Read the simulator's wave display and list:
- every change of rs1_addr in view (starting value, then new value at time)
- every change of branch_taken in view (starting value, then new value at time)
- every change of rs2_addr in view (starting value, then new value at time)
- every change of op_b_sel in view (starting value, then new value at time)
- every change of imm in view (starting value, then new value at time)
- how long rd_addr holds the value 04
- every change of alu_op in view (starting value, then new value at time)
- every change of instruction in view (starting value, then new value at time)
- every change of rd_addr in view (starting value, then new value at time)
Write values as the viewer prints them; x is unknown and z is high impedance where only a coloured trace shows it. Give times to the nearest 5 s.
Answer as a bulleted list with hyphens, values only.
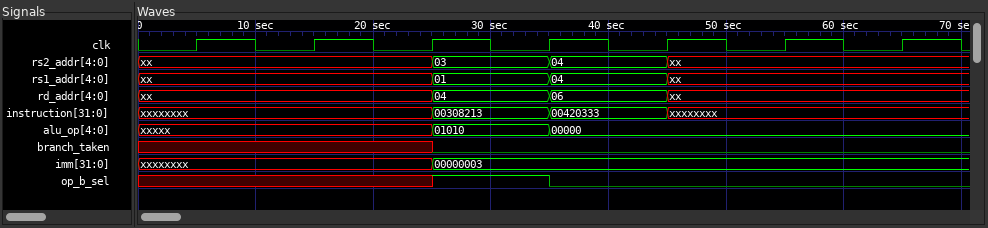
- xx, 01 at 25 s, 04 at 35 s, xx at 45 s
- x, 0 at 25 s
- xx, 03 at 25 s, 04 at 35 s, xx at 45 s
- x, 1 at 25 s, 0 at 35 s
- xxxxxxxx, 00000003 at 25 s
- 10 s
- xxxxx, 01010 at 25 s, 00000 at 35 s
- xxxxxxxx, 00308213 at 25 s, 00420333 at 35 s, xxxxxxxx at 45 s
- xx, 04 at 25 s, 06 at 35 s, xx at 45 s
